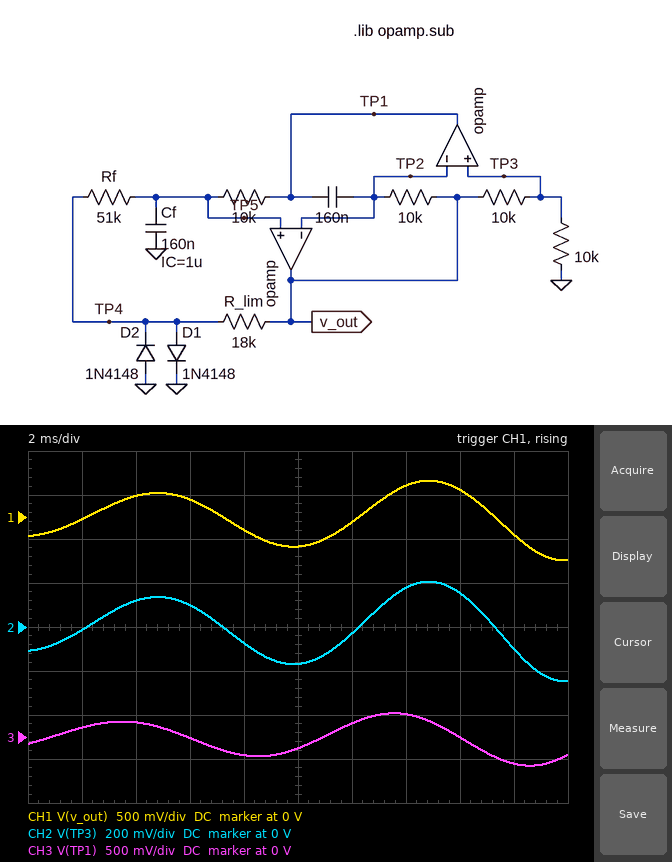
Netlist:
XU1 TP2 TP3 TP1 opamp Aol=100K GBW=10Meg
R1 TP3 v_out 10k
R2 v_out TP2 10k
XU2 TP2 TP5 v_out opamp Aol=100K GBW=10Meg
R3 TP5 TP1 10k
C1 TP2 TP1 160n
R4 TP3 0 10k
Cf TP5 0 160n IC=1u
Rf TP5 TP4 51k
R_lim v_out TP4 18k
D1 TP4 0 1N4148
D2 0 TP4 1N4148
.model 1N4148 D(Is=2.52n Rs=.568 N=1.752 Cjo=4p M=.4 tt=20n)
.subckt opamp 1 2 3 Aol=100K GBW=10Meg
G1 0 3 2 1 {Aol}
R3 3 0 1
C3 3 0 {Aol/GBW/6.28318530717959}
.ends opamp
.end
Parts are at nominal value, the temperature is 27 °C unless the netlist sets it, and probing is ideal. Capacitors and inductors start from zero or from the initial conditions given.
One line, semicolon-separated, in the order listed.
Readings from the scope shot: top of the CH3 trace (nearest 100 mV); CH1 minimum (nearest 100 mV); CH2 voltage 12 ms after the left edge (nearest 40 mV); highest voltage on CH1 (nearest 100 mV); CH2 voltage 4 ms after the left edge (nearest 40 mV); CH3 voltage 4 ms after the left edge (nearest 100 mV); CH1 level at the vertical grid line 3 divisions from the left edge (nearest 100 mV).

300 mV; -500 mV; -40 mV; 400 mV; 120 mV; 200 mV; 200 mV
